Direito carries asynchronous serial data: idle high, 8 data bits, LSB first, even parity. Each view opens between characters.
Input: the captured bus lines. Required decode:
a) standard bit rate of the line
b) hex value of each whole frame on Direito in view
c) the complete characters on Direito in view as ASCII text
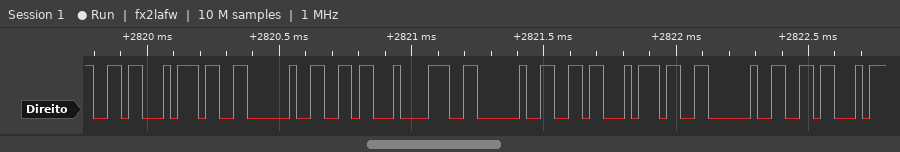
38400 baud
36, 37, 20, 36, 38, 20, 36, 37, 20, 36
"67 68 67 6"
